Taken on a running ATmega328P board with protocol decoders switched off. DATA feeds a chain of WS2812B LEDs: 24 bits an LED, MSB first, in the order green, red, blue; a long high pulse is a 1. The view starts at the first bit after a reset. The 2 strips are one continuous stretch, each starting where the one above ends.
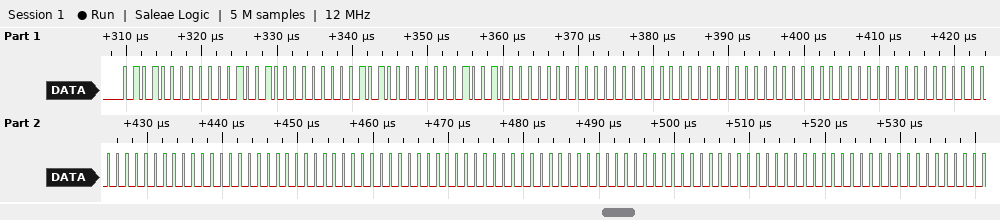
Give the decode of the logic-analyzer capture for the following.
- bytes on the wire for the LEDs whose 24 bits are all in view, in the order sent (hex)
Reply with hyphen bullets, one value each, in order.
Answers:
- 50 09 00 50 09 00 00 00 00 00 00 00 00 00 00 00 00 00 00 00 00
